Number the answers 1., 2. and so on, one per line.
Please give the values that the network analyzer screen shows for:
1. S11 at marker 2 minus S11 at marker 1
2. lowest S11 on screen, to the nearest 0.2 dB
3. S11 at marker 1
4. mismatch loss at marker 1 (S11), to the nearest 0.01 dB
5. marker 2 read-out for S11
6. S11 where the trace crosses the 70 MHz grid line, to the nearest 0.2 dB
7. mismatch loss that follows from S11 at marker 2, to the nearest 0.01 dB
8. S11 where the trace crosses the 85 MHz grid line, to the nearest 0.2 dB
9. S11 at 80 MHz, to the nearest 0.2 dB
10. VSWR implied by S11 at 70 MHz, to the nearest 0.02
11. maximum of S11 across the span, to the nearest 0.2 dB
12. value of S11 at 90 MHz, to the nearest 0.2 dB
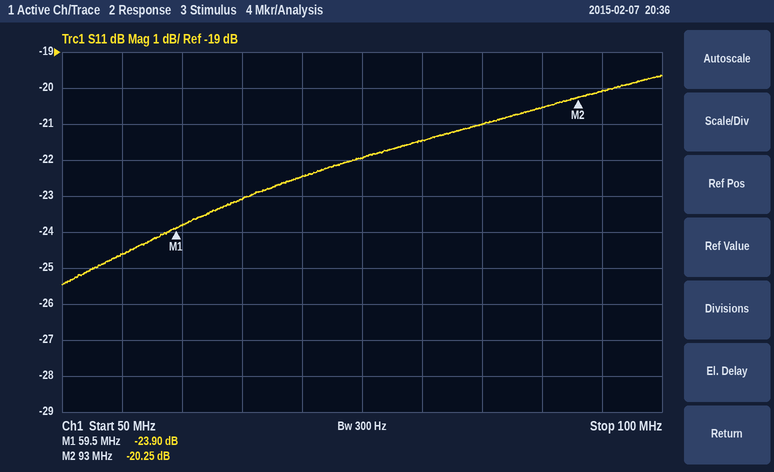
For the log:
1. 3.65 dB
2. -25.4 dB
3. -23.90 dB
4. 0.02 dB
5. -20.25 dB
6. -22.4 dB
7. 0.04 dB
8. -21.0 dB
9. -21.4 dB
10. 1.16
11. -19.6 dB
12. -20.6 dB
